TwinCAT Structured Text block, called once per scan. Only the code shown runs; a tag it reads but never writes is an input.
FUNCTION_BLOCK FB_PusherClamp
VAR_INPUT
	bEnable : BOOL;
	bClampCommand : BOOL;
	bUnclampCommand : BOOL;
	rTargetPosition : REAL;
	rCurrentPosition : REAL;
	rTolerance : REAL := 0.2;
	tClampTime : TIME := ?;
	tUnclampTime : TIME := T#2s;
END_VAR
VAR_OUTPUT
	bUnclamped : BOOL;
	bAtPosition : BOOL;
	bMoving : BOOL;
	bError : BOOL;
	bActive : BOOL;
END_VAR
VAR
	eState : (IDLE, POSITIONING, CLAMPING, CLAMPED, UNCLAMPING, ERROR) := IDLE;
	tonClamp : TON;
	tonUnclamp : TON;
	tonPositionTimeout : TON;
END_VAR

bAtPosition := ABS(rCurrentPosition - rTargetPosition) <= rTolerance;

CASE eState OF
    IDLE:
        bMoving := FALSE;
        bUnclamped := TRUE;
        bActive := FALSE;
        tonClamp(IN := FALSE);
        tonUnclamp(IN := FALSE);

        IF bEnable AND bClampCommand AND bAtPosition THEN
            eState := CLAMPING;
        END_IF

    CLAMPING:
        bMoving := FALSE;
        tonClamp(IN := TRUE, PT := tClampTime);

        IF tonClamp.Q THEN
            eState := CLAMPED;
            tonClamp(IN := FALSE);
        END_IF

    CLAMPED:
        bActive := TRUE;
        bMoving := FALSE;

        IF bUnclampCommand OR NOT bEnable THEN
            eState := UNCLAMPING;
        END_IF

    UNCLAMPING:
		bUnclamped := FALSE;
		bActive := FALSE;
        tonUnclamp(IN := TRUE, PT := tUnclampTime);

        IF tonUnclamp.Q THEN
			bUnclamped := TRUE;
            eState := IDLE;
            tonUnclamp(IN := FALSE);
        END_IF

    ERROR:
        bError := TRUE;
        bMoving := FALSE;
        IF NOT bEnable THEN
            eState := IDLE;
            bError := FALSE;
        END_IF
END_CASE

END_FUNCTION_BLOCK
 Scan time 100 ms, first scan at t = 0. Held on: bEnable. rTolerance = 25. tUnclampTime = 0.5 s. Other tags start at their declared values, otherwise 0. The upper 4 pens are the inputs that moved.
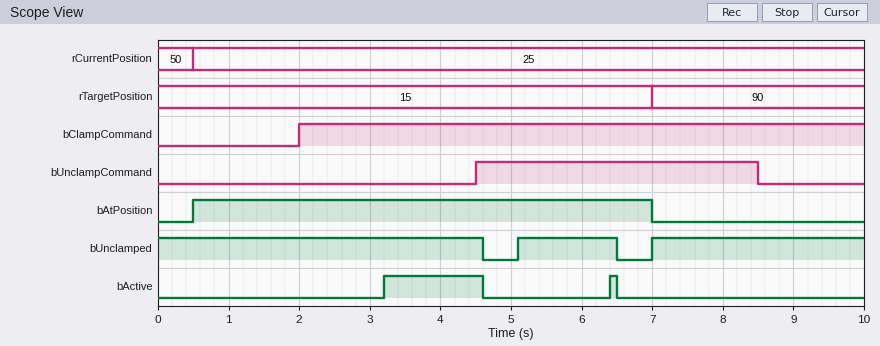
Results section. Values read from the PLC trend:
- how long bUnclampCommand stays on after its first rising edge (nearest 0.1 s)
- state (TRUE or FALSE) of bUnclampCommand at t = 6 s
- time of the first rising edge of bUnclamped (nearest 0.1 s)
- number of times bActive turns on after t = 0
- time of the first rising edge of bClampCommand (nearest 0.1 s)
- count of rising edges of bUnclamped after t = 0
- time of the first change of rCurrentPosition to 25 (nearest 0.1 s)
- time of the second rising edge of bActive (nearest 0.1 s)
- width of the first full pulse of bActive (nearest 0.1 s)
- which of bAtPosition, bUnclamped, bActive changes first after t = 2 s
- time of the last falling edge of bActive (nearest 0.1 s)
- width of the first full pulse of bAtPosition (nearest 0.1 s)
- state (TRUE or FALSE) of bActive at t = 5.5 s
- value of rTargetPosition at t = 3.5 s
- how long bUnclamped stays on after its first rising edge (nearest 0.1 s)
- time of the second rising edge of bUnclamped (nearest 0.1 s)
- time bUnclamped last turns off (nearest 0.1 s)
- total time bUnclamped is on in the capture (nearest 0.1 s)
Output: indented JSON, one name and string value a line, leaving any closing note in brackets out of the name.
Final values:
{
  "how long bUnclampCommand stays on after its first rising edge": "4.0 s",
  "state (TRUE or FALSE) of bUnclampCommand at t = 6 s": "TRUE",
  "time of the first rising edge of bUnclamped": "5.1 s",
  "number of times bActive turns on after t = 0": "2",
  "time of the first rising edge of bClampCommand": "2.0 s",
  "count of rising edges of bUnclamped after t = 0": "2",
  "time of the first change of rCurrentPosition to 25": "0.5 s",
  "time of the second rising edge of bActive": "6.4 s",
  "width of the first full pulse of bActive": "1.4 s",
  "which of bAtPosition, bUnclamped, bActive changes first after t = 2 s": "bActive",
  "time of the last falling edge of bActive": "6.5 s",
  "width of the first full pulse of bAtPosition": "6.5 s",
  "state (TRUE or FALSE) of bActive at t = 5.5 s": "FALSE",
  "value of rTargetPosition at t = 3.5 s": "15",
  "how long bUnclamped stays on after its first rising edge": "1.4 s",
  "time of the second rising edge of bUnclamped": "7.0 s",
  "time bUnclamped last turns off": "6.5 s",
  "total time bUnclamped is on in the capture": "9.0 s"
}
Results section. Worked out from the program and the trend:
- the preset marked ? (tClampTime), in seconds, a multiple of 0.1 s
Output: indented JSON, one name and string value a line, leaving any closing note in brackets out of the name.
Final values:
{
  "the preset marked ? (tClampTime), in seconds, a multiple of 0.1 s": "1.0 s"
}
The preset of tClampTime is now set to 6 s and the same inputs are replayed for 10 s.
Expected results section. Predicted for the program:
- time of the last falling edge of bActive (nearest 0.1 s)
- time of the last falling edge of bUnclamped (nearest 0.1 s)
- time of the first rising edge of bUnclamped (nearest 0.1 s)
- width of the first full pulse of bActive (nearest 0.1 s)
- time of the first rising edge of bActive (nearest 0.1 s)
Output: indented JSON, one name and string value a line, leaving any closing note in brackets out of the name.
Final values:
{
  "time of the last falling edge of bActive": "8.3 s",
  "time of the last falling edge of bUnclamped": "8.3 s",
  "time of the first rising edge of bUnclamped": "8.8 s",
  "width of the first full pulse of bActive": "0.1 s",
  "time of the first rising edge of bActive": "8.2 s"
}
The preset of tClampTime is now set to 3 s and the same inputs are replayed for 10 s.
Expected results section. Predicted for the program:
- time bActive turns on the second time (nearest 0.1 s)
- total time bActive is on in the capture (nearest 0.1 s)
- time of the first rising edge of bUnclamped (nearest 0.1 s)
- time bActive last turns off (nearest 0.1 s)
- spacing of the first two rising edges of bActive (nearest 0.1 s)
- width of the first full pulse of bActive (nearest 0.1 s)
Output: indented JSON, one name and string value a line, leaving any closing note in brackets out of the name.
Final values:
{
  "time bActive turns on the second time": "9.1 s",
  "total time bActive is on in the capture": "1.0 s",
  "time of the first rising edge of bUnclamped": "5.8 s",
  "time bActive last turns off": "5.3 s",
  "spacing of the first two rising edges of bActive": "3.9 s",
  "width of the first full pulse of bActive": "0.1 s"
}
